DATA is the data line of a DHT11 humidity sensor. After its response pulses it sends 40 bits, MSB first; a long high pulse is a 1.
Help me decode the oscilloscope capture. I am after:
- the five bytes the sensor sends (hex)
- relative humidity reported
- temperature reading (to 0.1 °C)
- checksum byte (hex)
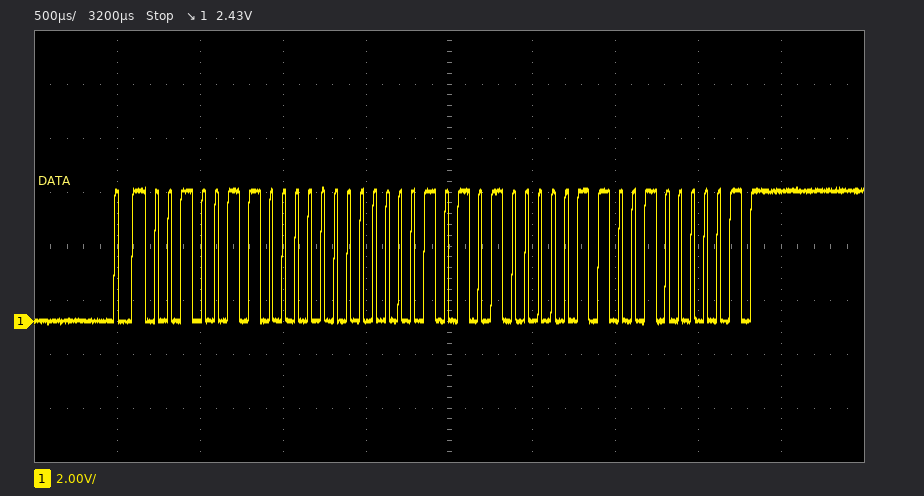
26 00 15 06 41
38 %
21.6 °C
0x41
